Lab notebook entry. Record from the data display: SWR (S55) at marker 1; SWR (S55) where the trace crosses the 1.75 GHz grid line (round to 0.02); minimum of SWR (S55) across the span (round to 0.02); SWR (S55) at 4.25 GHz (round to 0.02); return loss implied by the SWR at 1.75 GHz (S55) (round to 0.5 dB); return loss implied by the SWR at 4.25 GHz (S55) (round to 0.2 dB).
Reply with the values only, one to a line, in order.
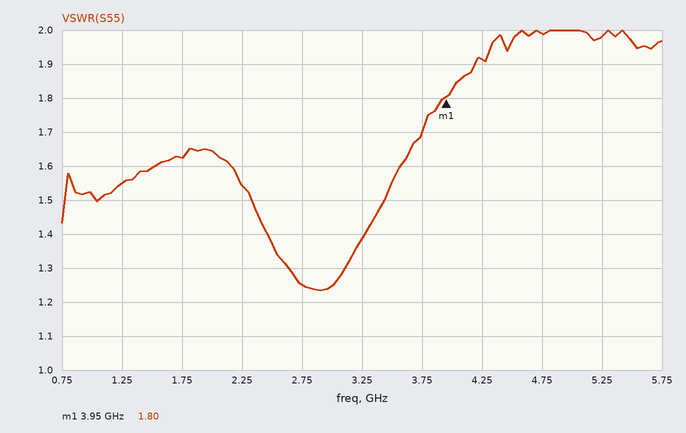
1.80
1.62
1.24
1.92
12.5 dB
10.0 dB
